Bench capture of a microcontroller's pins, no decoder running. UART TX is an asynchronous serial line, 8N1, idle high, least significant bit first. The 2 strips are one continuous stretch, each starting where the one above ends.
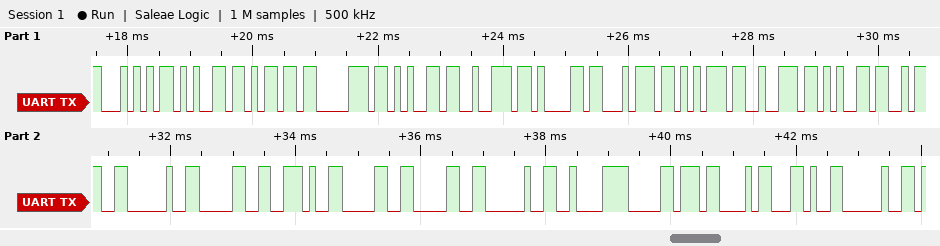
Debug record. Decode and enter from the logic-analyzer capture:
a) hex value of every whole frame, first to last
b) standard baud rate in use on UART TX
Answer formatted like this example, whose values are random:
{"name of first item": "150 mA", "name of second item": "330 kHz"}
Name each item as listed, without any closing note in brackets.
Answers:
{"hex value of every whole frame, first to last": "54 65 6D 70 65 72 61 74 75 72 65 3A 20 30 2E 30 30 20 C2 B0 43 2C 20", "standard baud rate in use on UART TX": "9600 baud"}
